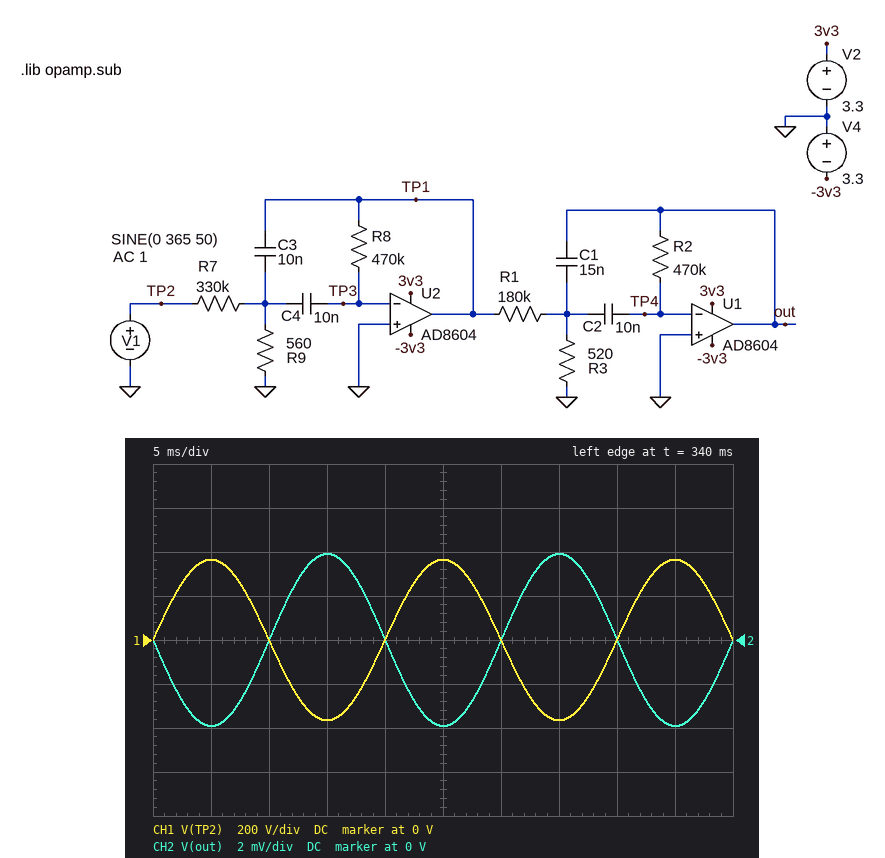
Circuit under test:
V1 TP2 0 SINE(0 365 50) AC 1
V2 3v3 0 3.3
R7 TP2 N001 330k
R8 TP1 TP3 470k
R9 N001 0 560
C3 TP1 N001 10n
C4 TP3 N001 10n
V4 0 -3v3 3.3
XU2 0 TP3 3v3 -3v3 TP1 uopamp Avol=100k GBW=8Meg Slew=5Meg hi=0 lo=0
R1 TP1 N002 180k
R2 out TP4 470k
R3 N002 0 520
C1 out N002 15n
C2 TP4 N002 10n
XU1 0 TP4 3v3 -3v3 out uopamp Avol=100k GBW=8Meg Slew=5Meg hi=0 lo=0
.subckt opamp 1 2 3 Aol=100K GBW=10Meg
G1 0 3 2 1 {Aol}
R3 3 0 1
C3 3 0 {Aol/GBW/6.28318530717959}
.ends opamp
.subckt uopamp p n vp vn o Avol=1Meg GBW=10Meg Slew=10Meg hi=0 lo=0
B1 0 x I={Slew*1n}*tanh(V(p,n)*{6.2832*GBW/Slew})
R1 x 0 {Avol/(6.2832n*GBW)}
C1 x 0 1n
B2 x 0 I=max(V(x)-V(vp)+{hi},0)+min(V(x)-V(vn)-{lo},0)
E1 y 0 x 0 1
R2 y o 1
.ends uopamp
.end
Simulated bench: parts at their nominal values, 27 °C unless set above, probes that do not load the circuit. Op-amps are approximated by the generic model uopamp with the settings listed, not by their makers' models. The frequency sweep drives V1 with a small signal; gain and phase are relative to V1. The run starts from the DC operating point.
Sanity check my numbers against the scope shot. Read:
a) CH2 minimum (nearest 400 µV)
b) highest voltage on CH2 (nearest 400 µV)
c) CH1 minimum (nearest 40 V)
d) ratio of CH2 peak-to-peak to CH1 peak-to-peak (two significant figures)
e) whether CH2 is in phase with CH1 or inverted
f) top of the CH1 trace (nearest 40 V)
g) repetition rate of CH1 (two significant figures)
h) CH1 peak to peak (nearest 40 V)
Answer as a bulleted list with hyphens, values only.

- -4.0 mV
- 4.0 mV
- -360 V
- 0.000011
- inverted
- 360 V
- 50 Hz
- 720 V
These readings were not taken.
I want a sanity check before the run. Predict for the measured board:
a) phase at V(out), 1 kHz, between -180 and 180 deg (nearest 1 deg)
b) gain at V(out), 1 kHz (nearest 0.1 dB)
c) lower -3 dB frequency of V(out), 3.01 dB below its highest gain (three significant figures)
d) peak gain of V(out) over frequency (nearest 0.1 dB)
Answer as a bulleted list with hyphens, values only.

- -110 deg
- -18.8 dB
- 812 Hz
- -16.2 dB
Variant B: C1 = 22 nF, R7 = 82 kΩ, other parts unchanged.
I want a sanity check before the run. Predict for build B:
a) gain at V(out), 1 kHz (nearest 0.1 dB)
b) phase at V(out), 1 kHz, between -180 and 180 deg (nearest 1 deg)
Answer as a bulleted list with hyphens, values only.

- -14.3 dB
- -112 deg
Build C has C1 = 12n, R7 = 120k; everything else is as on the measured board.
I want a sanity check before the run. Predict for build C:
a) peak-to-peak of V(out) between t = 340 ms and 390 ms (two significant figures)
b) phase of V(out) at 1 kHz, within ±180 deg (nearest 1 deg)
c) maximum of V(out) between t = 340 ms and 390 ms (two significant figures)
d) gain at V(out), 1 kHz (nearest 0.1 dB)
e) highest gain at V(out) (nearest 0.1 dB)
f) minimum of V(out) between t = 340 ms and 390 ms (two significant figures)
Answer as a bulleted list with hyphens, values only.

- 21 mV
- -94 deg
- 11 mV
- -1.5 dB
- 2.9 dB
- -11 mV
